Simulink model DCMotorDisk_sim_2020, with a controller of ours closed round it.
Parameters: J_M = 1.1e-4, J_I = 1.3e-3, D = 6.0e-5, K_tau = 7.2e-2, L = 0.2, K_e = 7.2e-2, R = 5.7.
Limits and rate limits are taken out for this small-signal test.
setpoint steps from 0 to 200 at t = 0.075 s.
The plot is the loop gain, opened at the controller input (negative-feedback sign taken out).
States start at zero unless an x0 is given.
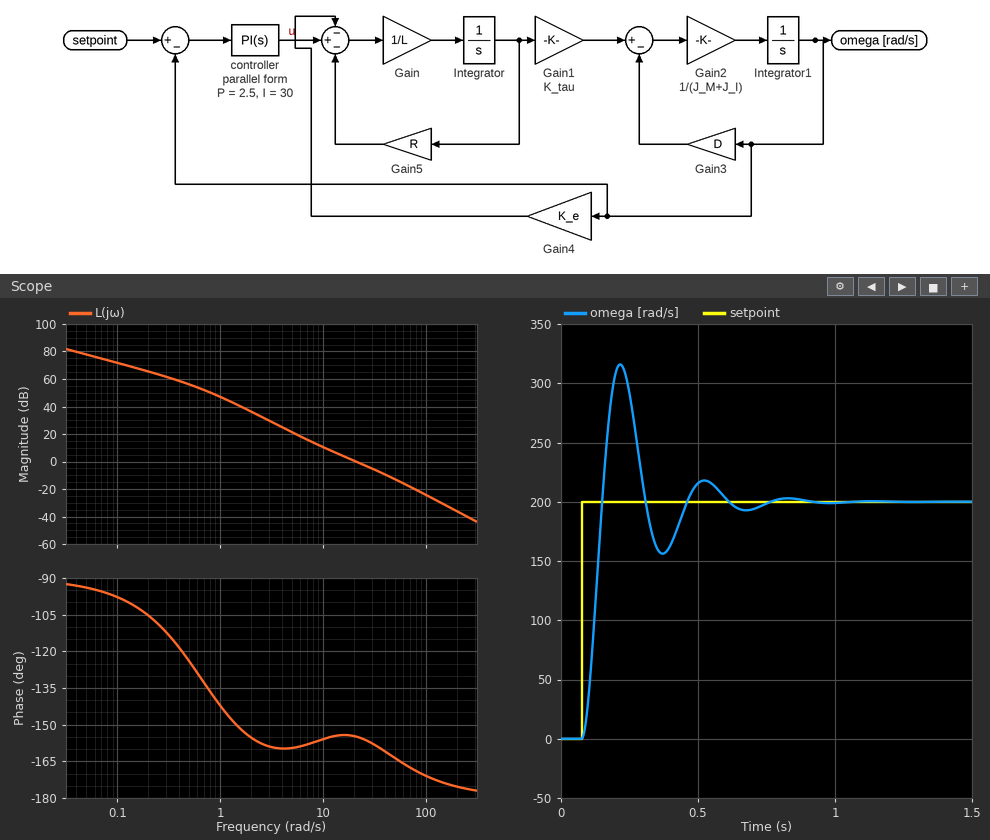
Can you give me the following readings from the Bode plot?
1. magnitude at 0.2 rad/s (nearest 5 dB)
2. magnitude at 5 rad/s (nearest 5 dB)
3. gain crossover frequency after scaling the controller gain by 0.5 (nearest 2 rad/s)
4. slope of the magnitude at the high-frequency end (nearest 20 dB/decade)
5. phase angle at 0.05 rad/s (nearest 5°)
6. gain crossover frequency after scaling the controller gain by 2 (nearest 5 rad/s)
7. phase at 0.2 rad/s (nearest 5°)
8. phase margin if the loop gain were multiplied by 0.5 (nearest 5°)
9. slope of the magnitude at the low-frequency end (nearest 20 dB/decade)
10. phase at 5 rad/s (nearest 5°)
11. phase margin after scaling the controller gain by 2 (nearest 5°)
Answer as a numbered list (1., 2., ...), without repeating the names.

1. 65 dB
2. 20 dB
3. 14 rad/s
4. -40 dB/decade
5. -95°
6. 30 rad/s
7. -105°
8. 25°
9. -20 dB/decade
10. -160°
11. 20°
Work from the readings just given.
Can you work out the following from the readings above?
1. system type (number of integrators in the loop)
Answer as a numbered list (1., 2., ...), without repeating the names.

1. 1
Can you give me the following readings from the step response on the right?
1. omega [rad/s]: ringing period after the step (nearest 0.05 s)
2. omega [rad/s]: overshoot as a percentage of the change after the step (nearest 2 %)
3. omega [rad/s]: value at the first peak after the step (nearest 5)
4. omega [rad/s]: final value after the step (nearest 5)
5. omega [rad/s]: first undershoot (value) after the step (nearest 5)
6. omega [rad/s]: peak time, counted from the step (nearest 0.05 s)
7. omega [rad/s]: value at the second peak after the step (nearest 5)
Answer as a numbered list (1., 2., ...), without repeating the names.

1. 0.30 s
2. 58 %
3. 315
4. 200
5. 155
6. 0.15 s
7. 220
